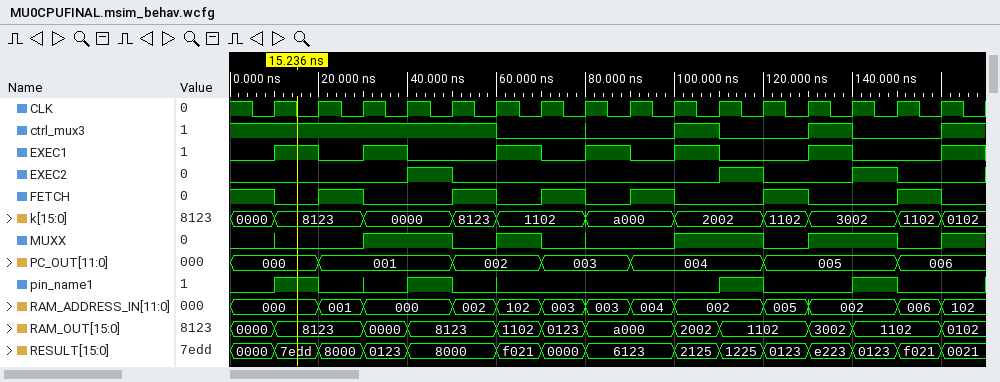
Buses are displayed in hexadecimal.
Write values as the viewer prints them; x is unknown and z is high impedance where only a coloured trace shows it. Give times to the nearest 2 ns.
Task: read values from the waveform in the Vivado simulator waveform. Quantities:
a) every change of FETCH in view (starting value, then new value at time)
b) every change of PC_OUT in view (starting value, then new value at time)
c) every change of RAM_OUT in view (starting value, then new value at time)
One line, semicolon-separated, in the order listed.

1, 0 at 10 ns, 1 at 20 ns, 0 at 30 ns, 1 at 50 ns, 0 at 60 ns, 1 at 70 ns, 0 at 80 ns, 1 at 90 ns, 0 at 100 ns, 1 at 120 ns, 0 at 130 ns, 1 at 150 ns, 0 at 160 ns; 000, 001 at 20 ns, 002 at 50 ns, 003 at 70 ns, 004 at 90 ns, 005 at 120 ns, 006 at 150 ns; 0000, 8123 at 10 ns, 0000 at 30 ns, 8123 at 40 ns, 1102 at 60 ns, 0123 at 70 ns, a000 at 80 ns, 2002 at 100 ns, 1102 at 110 ns, 3002 at 130 ns, 1102 at 140 ns, 0102 at 160 ns
